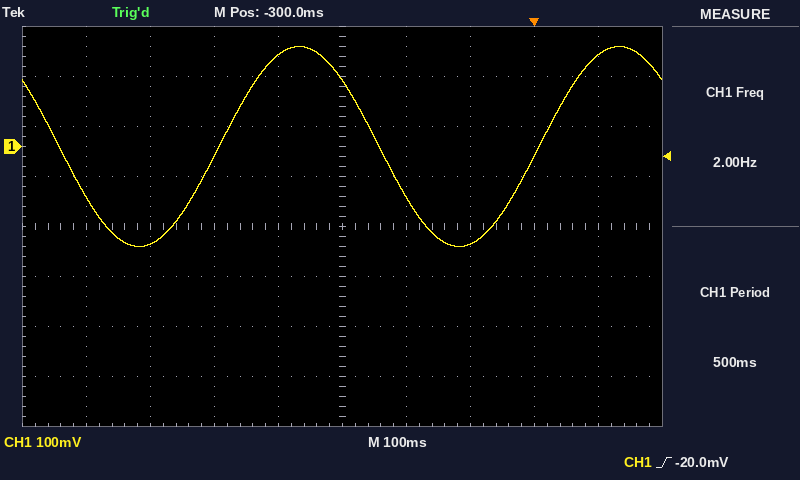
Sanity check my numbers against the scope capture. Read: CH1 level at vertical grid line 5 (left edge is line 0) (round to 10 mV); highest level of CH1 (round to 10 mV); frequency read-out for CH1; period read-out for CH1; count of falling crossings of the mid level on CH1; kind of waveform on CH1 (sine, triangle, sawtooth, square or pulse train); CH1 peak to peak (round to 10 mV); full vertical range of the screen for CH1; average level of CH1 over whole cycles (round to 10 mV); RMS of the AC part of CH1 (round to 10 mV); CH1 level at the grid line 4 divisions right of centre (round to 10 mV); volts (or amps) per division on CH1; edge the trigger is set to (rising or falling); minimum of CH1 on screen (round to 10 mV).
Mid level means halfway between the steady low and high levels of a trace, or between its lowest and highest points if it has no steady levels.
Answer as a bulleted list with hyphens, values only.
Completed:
- 130 mV
- 200 mV
- 2.00 Hz
- 500 ms
- 2
- sine
- 400 mV
- 800 mV
- 0 mV
- 140 mV
- 180 mV
- 100 mV
- rising
- -200 mV
